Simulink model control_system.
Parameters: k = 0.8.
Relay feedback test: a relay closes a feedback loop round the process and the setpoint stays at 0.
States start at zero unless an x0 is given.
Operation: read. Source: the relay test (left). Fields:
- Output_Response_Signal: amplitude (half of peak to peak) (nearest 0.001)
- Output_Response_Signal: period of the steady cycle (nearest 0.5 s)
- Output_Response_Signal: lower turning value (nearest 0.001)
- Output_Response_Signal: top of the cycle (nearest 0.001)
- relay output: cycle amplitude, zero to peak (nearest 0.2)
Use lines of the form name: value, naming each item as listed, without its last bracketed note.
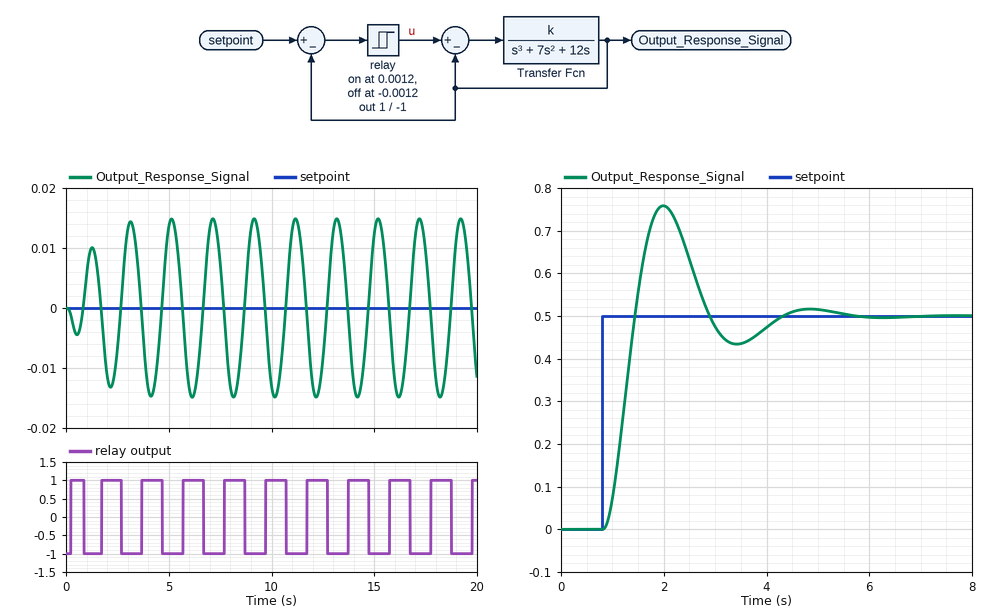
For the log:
Output_Response_Signal: amplitude (half of peak to peak): 0.015
Output_Response_Signal: period of the steady cycle: 2.0 s
Output_Response_Signal: lower turning value: -0.015
Output_Response_Signal: top of the cycle: 0.015
relay output: cycle amplitude, zero to peak: 1.0
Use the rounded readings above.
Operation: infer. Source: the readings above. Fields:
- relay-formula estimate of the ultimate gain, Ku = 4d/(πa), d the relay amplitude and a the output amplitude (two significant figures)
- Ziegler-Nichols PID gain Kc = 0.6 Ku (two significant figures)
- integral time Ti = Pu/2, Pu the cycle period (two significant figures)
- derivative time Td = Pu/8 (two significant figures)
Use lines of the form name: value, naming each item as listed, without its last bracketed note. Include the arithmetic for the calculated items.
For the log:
relay-formula estimate of the ultimate gain, Ku = 4d/(πa), d the relay amplitude and a the output amplitude: 4 × 1 / (π × 0.015) = 85
Ziegler-Nichols PID gain Kc = 0.6 Ku: 0.6 × 85 = 51
integral time Ti = Pu/2, Pu the cycle period: 2 / 2 = 1.0 s
derivative time Td = Pu/8: 2 / 8 = 0.25 s
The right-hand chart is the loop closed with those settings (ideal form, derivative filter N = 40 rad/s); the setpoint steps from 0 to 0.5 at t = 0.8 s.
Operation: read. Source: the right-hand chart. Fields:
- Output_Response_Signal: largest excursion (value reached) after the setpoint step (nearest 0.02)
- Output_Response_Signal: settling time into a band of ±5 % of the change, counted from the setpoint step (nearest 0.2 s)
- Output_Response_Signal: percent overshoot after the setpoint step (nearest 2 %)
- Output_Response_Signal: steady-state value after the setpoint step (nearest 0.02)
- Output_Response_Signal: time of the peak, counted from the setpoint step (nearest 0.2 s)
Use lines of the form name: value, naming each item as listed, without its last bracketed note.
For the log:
Output_Response_Signal: largest excursion (value reached) after the setpoint step: 0.76
Output_Response_Signal: settling time into a band of ±5 % of the change, counted from the setpoint step: 3.2 s
Output_Response_Signal: percent overshoot after the setpoint step: 52 %
Output_Response_Signal: steady-state value after the setpoint step: 0.50
Output_Response_Signal: time of the peak, counted from the setpoint step: 1.2 s
